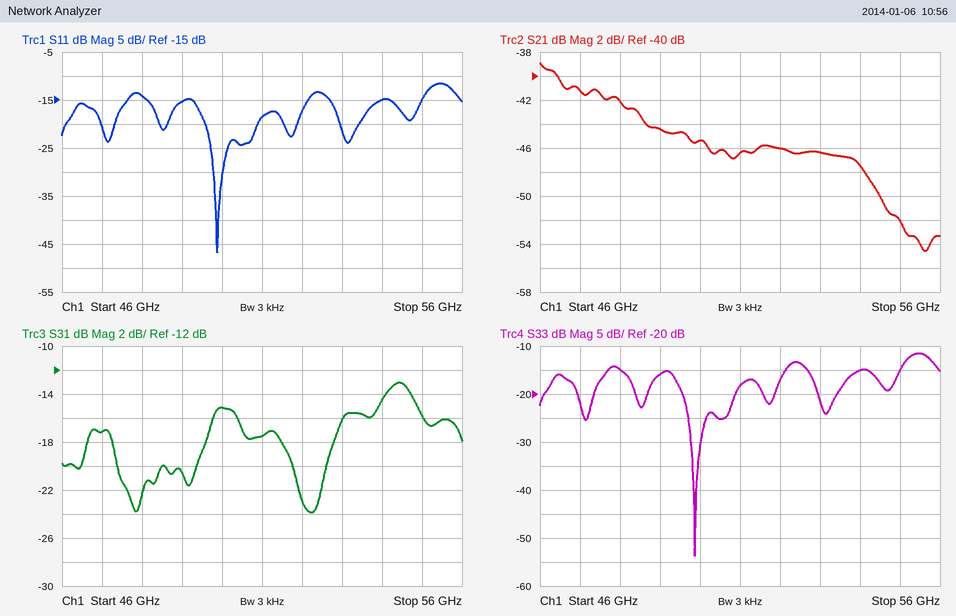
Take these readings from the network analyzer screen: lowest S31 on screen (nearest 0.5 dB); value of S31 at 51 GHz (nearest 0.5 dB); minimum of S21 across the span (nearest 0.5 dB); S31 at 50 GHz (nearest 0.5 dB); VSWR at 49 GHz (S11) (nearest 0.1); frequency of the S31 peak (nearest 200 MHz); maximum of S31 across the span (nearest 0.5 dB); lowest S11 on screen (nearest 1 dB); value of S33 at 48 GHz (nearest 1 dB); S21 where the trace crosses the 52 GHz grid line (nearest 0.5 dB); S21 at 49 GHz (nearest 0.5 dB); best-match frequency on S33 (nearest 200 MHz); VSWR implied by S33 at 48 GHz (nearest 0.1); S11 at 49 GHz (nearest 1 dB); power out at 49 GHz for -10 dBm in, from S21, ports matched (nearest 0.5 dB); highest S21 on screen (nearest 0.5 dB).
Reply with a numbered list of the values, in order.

1. -24.0 dB
2. -17.5 dB
3. -54.5 dB
4. -15.0 dB
5. 1.4
6. 54.4 GHz
7. -13.0 dB
8. -47 dB
9. -15 dB
10. -46.0 dB
11. -44.5 dB
12. 49.8 GHz
13. 1.4
14. -15 dB
15. -54.5 dBm
16. -39.0 dB
